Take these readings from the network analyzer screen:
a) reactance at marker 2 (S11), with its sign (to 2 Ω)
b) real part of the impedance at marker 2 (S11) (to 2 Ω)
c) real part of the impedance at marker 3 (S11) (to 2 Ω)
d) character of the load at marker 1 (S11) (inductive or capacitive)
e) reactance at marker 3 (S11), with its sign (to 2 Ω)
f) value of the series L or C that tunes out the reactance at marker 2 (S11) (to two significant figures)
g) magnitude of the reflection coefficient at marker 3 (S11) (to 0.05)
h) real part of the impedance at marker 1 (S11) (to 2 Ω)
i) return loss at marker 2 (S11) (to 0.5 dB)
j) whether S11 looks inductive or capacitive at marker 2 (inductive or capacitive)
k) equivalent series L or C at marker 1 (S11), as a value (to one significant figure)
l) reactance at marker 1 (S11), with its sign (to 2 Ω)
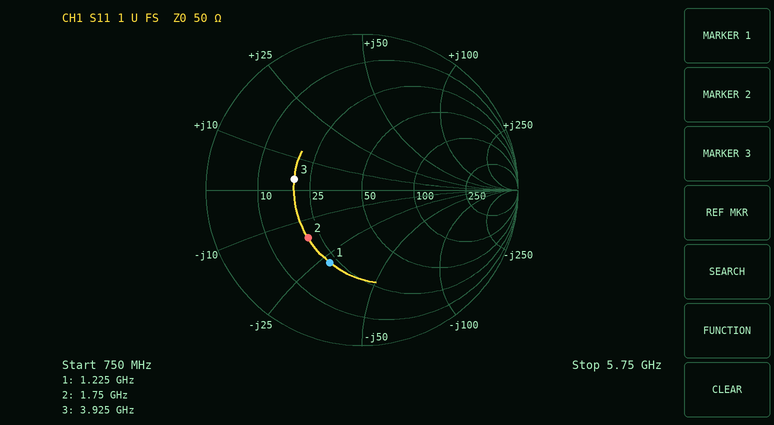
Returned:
-16 Ω
20 Ω
20 Ω
capacitive
+4 Ω
1.5 nH
0.45
22 Ω
6.5 dB
capacitive
5 pF
-28 Ω
